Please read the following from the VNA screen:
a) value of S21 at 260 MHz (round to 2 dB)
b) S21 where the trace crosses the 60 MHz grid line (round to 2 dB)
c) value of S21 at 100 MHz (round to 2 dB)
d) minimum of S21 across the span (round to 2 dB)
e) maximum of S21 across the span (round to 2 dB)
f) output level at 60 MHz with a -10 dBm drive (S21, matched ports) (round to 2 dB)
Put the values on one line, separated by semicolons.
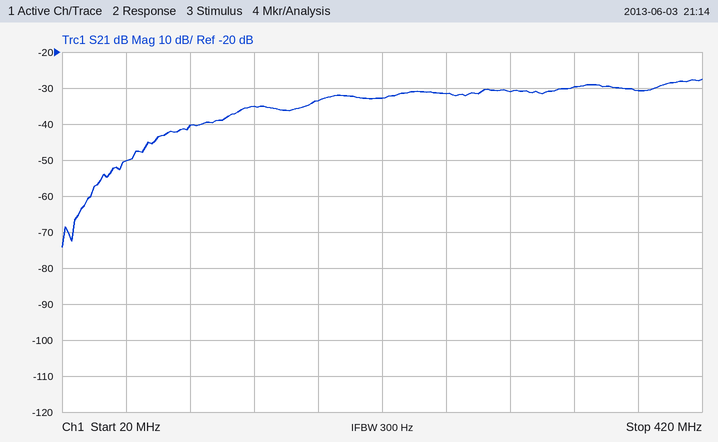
-32 dB; -50 dB; -40 dB; -74 dB; -28 dB; -60 dBm
